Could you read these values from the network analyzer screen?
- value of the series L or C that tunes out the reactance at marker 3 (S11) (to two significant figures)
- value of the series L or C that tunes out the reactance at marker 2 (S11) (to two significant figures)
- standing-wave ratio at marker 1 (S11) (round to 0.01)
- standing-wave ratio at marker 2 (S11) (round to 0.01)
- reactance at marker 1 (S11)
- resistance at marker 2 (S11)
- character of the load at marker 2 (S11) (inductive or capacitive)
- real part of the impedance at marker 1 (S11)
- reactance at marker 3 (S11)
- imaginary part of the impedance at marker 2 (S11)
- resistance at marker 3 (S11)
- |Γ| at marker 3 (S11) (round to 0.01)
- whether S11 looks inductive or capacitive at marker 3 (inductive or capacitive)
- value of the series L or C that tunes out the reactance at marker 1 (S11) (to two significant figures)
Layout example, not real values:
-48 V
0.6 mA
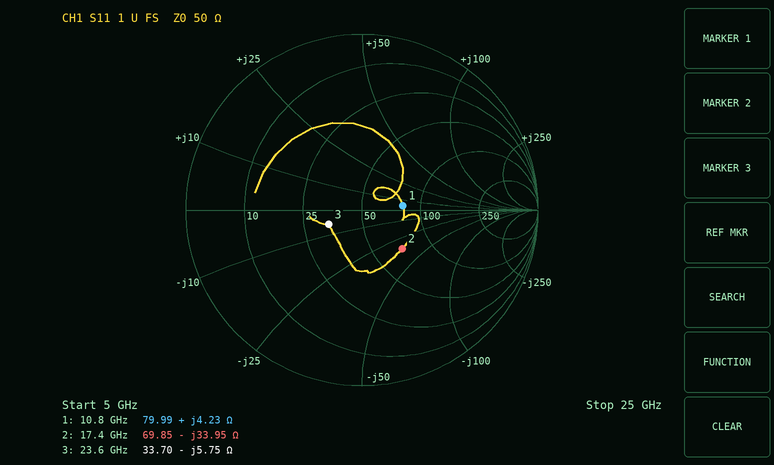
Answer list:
39 pH
310 pH
1.61
1.92
+4.23 Ω
69.85 Ω
capacitive
79.99 Ω
-5.75 Ω
-33.95 Ω
33.70 Ω
0.21
capacitive
3.5 pF
